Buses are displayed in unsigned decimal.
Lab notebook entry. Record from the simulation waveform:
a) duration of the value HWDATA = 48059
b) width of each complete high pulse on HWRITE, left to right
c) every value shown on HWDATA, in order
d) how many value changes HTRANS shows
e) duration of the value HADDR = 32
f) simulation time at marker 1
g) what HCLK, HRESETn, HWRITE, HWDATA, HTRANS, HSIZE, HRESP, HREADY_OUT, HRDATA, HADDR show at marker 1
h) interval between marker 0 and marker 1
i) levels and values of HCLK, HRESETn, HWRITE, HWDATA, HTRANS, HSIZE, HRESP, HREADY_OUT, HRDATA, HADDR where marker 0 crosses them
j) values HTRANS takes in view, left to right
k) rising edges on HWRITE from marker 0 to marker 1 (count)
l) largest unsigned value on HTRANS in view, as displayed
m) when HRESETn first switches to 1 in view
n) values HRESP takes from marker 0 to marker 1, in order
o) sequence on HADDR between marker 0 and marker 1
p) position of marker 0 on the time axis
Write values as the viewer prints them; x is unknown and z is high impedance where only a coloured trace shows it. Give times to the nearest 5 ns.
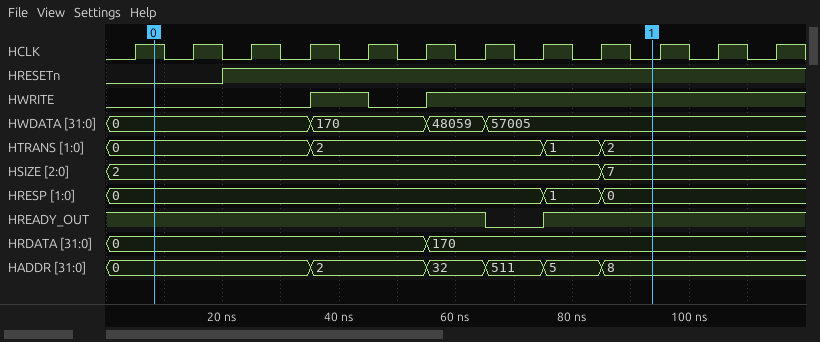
10 ns
10 ns
0, 170, 48059, 57005
3
10 ns
95 ns
HCLK=0, HRESETn=1, HWRITE=1, HWDATA=57005, HTRANS=2, HSIZE=7, HRESP=0, HREADY_OUT=1, HRDATA=170, HADDR=8
85 ns
HCLK=1, HRESETn=0, HWRITE=0, HWDATA=0, HTRANS=0, HSIZE=2, HRESP=0, HREADY_OUT=1, HRDATA=0, HADDR=0
0, 2, 1, 2
2
2
20 ns
0, 1, 0
0, 2, 32, 511, 5, 8
10 ns
